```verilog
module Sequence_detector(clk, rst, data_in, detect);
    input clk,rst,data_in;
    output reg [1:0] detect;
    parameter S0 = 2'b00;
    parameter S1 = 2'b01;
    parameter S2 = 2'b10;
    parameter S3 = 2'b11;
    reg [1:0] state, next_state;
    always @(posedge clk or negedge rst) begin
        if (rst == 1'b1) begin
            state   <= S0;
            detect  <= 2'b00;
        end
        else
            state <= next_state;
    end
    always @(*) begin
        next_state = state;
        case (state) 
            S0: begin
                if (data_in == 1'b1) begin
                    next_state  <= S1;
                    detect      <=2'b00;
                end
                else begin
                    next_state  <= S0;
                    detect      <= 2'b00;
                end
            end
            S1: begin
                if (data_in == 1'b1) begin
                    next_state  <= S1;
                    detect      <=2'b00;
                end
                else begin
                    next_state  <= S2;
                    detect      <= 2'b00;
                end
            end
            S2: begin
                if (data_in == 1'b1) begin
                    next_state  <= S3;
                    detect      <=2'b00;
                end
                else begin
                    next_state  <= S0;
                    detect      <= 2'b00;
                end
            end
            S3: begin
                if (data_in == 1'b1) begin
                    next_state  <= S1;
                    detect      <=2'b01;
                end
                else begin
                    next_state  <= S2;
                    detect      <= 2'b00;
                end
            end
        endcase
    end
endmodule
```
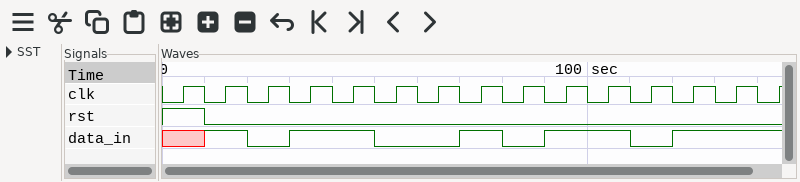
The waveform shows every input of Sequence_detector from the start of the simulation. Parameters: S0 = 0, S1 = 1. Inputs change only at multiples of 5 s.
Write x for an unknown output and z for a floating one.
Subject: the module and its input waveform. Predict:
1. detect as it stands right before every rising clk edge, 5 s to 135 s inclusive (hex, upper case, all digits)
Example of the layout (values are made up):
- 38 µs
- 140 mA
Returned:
- x, 0, 0, 0, 1, 0, 0, 0, 0, 0, 1, 0, 0, 1
